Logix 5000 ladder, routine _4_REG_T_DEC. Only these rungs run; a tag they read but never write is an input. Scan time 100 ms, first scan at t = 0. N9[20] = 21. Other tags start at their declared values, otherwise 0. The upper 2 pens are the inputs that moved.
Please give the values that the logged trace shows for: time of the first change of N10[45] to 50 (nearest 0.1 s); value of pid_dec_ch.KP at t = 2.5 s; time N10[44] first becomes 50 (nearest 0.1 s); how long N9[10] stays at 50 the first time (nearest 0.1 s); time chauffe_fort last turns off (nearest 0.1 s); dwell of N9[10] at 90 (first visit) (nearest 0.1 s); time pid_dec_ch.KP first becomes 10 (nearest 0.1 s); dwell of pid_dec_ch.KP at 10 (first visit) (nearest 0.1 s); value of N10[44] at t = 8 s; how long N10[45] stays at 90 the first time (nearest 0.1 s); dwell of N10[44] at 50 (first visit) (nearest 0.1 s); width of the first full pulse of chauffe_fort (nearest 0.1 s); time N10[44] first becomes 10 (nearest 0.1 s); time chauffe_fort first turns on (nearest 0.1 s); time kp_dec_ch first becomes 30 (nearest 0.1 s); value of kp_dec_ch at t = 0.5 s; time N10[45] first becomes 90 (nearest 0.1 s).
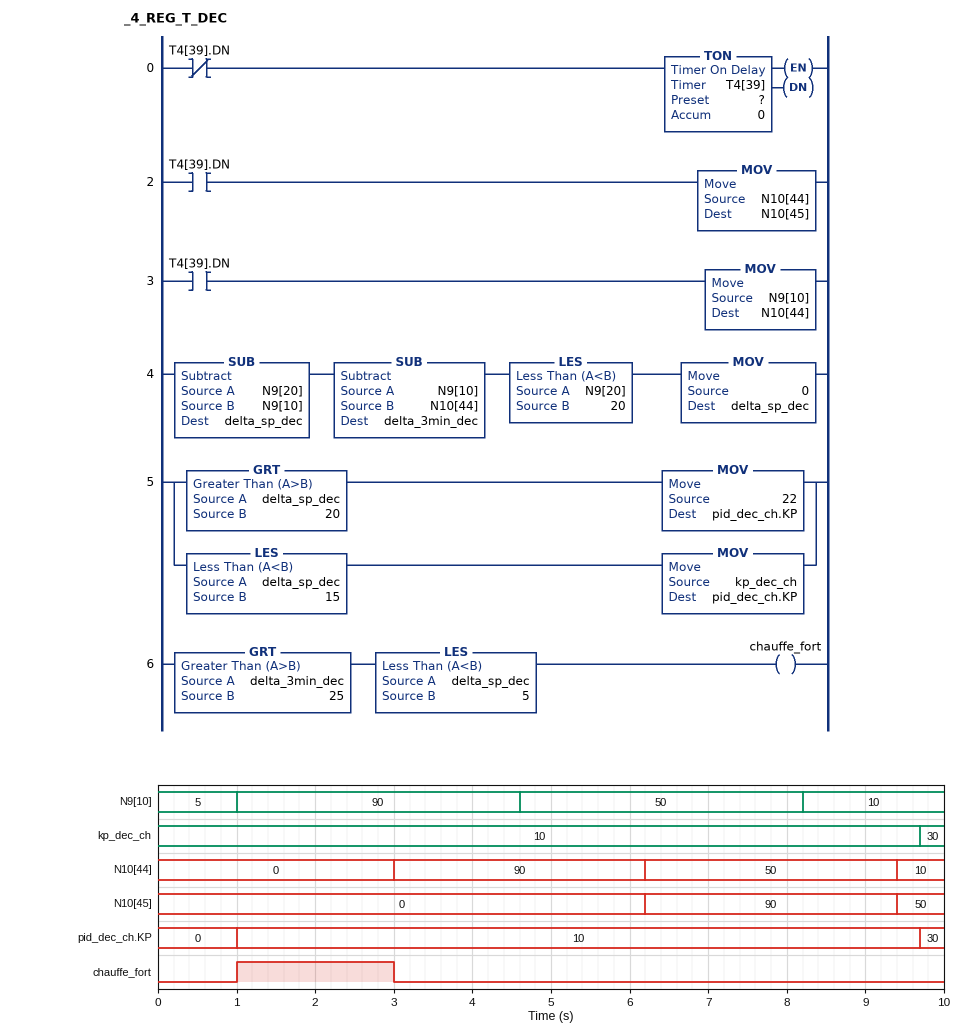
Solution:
9.4 s
10
6.2 s
3.6 s
3.0 s
3.6 s
1.0 s
8.7 s
50
3.2 s
3.2 s
2.0 s
9.4 s
1.0 s
9.7 s
10
6.2 s
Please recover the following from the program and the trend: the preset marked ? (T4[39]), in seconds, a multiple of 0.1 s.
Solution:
3.0 s
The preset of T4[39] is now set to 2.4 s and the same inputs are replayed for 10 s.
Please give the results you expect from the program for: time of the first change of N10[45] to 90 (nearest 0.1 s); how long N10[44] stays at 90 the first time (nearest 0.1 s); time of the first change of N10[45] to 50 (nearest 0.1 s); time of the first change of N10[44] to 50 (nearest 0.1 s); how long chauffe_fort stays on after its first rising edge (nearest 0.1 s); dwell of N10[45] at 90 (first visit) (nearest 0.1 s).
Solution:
5.0 s
2.6 s
7.6 s
5.0 s
1.4 s
2.6 s
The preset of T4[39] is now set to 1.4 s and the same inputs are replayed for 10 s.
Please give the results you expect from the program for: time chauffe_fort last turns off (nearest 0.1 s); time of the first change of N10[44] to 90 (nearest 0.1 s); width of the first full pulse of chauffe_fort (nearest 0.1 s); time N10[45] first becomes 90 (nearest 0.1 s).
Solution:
1.4 s
1.4 s
0.4 s
3.0 s
